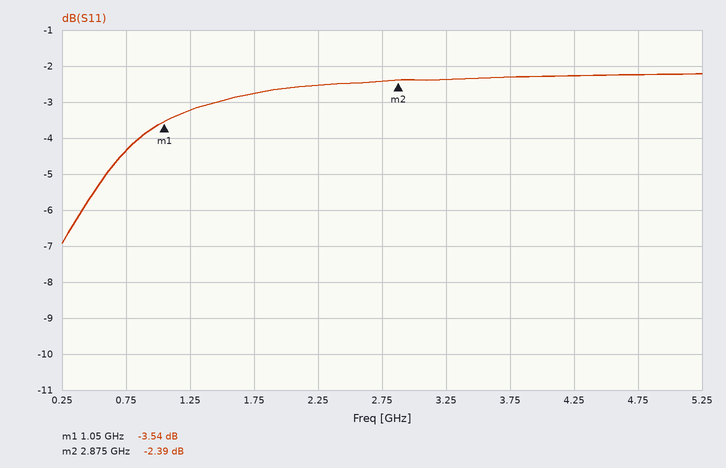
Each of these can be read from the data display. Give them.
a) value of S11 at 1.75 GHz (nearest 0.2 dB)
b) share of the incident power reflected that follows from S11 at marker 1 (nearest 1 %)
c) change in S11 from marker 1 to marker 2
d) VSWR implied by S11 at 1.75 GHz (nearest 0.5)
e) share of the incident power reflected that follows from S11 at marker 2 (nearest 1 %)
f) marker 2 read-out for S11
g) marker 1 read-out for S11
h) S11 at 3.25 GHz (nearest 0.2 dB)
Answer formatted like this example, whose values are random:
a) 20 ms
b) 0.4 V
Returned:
a) -2.8 dB
b) 44 %
c) 1.15 dB
d) 6.5
e) 58 %
f) -2.39 dB
g) -3.54 dB
h) -2.4 dB
